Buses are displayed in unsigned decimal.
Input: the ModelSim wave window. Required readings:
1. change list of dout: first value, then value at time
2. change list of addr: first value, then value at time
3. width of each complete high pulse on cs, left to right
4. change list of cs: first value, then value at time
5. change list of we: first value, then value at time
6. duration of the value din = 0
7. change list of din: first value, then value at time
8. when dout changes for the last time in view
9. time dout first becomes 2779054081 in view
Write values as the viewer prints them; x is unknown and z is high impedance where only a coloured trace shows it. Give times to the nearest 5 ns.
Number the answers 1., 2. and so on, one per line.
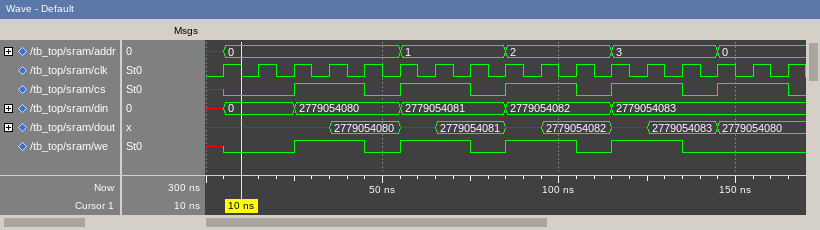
1. x, 2779054080 at 35 ns, x at 55 ns, 2779054081 at 65 ns, x at 85 ns, 2779054082 at 95 ns, x at 115 ns, 2779054083 at 125 ns, 2779054080 at 145 ns
2. x, 0 at 5 ns, 1 at 55 ns, 2 at 85 ns, 3 at 115 ns, 0 at 145 ns
3. 20 ns, 20 ns, 20 ns, 20 ns, 20 ns
4. x, 0 at 5 ns, 1 at 25 ns, 0 at 45 ns, 1 at 55 ns, 0 at 75 ns, 1 at 85 ns, 0 at 105 ns, 1 at 115 ns, 0 at 135 ns, 1 at 145 ns, 0 at 165 ns
5. x, 0 at 5 ns, 1 at 25 ns, 0 at 45 ns, 1 at 55 ns, 0 at 75 ns, 1 at 85 ns, 0 at 105 ns, 1 at 115 ns, 0 at 135 ns
6. 20 ns
7. x, 0 at 5 ns, 2779054080 at 25 ns, 2779054081 at 55 ns, 2779054082 at 85 ns, 2779054083 at 115 ns
8. 145 ns
9. 65 ns
